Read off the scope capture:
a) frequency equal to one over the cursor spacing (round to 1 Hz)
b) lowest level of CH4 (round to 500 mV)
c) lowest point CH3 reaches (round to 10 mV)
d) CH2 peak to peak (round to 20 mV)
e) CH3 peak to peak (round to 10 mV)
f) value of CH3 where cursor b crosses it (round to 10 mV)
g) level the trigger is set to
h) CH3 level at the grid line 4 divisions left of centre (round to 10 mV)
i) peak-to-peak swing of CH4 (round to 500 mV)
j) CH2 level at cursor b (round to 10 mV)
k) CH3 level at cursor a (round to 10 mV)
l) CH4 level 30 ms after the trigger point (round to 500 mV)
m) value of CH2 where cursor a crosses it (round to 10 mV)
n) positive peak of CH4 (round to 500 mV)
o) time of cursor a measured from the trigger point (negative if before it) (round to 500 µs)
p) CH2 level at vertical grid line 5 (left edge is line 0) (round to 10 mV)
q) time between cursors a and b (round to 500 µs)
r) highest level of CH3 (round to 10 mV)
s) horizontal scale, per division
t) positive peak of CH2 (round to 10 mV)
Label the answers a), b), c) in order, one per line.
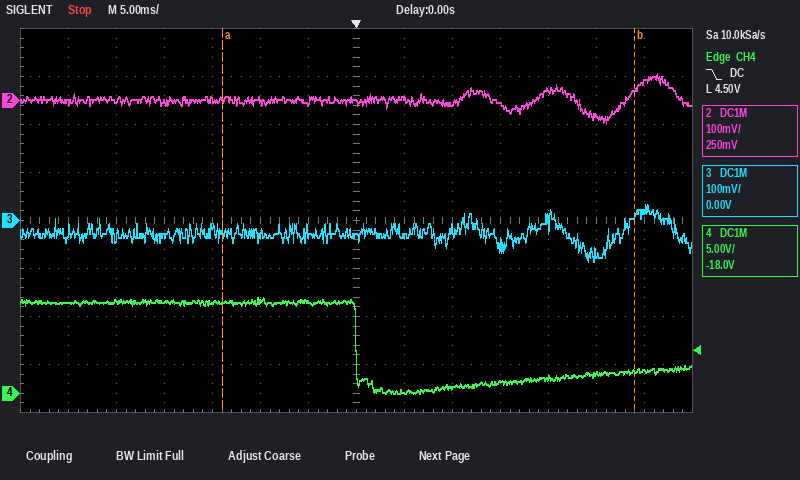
a) 23 Hz
b) 0.0 V
c) -90 mV
d) 100 mV
e) 120 mV
f) 10 mV
g) 4.50 V
h) -30 mV
i) 10.0 V
j) 20 mV
k) -30 mV
l) 2.5 V
m) 0 mV
n) 10.0 V
o) -14.0 ms
p) 0 mV
q) 43.0 ms
r) 30 mV
s) 5 ms
t) 60 mV
